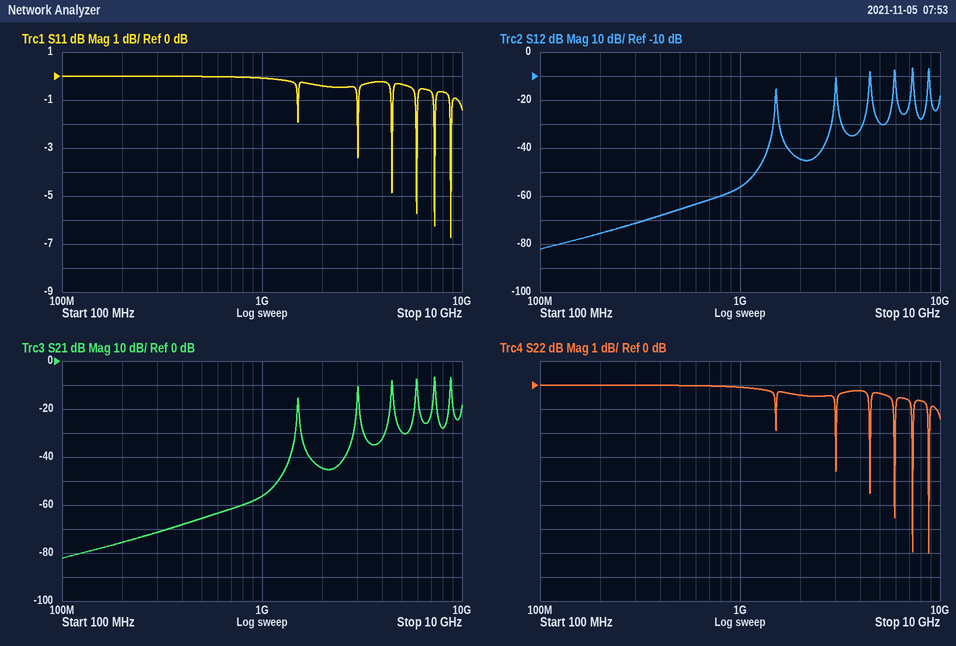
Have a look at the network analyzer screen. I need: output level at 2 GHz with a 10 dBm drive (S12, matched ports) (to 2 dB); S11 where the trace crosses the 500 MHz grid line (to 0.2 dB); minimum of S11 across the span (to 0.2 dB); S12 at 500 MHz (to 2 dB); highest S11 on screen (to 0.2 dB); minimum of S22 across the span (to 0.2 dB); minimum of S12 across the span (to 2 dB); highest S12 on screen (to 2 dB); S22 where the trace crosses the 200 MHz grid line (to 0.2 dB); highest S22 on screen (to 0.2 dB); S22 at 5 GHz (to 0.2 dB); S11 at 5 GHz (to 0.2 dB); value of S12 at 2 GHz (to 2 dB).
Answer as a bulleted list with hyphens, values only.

- -34 dBm
- 0.0 dB
- -6.8 dB
- -66 dB
- 0.0 dB
- -7.0 dB
- -82 dB
- -6 dB
- 0.0 dB
- 0.0 dB
- -0.4 dB
- -0.4 dB
- -44 dB
